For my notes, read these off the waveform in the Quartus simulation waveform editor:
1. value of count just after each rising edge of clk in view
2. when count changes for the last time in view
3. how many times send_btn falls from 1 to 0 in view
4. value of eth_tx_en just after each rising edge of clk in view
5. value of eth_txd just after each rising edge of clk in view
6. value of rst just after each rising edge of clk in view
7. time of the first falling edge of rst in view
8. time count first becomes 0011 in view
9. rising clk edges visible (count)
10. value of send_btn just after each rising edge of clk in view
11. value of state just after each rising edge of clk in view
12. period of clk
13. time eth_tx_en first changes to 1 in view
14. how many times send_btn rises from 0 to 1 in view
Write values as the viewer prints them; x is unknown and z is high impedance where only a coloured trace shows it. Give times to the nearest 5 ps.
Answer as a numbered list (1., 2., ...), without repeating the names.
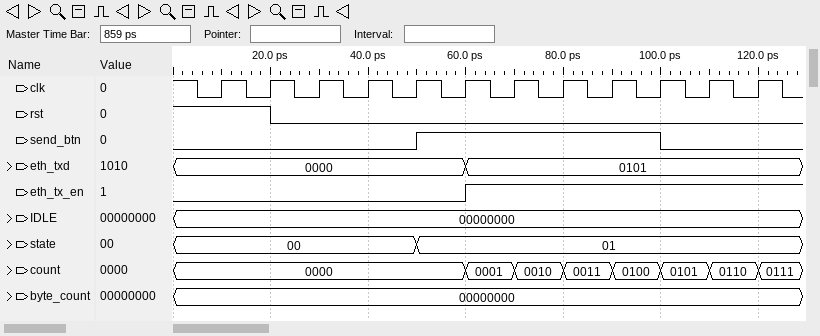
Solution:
1. 0000, 0000, 0000, 0000, 0000, 0001, 0010, 0011, 0100, 0101, 0110, 0111
2. 120 ps
3. 1
4. 0 0 0 0 0 1 1 1 1 1 1 1
5. 0000, 0000, 0000, 0000, 0000, 0101, 0101, 0101, 0101, 0101, 0101, 0101
6. 1 0 0 0 0 0 0 0 0 0 0 0
7. 20 ps
8. 80 ps
9. 12
10. 0 0 0 0 1 1 1 1 1 0 0 0
11. 00, 00, 00, 00, 01, 01, 01, 01, 01, 01, 01, 01
12. 10 ps
13. 60 ps
14. 1
